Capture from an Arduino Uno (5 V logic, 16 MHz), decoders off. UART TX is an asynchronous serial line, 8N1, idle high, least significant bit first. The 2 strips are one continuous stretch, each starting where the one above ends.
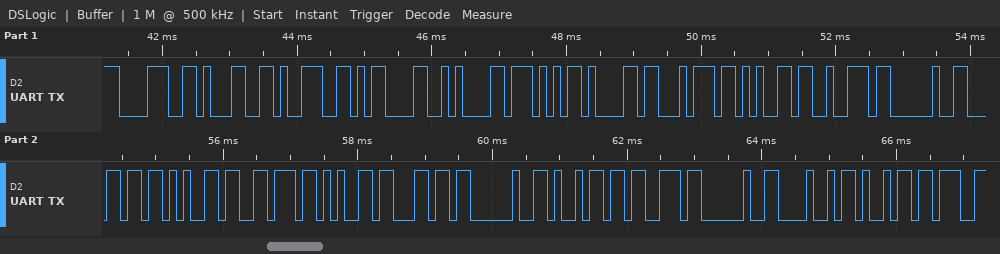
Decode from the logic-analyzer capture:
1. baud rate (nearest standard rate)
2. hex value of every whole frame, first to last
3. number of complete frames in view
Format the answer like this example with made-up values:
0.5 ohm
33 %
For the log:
9600 baud
38 31 39 0D 0A 57 61 74 65 72 20 6C 65 76 65 6C 20 69 73 20 48 69
22
